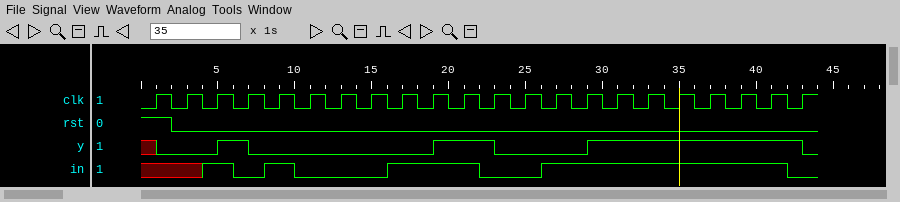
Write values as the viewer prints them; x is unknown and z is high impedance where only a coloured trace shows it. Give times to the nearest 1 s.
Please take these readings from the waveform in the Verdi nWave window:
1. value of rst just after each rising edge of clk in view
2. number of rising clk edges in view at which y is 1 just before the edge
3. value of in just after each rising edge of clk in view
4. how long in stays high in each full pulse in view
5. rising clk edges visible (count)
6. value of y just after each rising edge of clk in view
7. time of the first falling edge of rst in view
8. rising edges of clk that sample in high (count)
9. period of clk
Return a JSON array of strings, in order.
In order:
["1 0 0 0 0 0 0 0 0 0 0 0 0 0 0 0 0 0 0 0 0 0", "10", "x x 1 0 1 0 0 0 1 1 1 0 0 1 1 1 1 1 1 1 1 0", "2 s, 6 s, 16 s", "22", "0 0 1 0 0 0 0 0 0 1 1 0 0 0 1 1 1 1 1 1 1 0", "2 s", "13", "2 s"]
